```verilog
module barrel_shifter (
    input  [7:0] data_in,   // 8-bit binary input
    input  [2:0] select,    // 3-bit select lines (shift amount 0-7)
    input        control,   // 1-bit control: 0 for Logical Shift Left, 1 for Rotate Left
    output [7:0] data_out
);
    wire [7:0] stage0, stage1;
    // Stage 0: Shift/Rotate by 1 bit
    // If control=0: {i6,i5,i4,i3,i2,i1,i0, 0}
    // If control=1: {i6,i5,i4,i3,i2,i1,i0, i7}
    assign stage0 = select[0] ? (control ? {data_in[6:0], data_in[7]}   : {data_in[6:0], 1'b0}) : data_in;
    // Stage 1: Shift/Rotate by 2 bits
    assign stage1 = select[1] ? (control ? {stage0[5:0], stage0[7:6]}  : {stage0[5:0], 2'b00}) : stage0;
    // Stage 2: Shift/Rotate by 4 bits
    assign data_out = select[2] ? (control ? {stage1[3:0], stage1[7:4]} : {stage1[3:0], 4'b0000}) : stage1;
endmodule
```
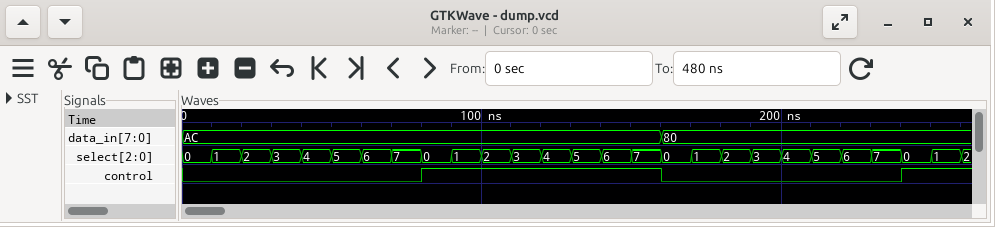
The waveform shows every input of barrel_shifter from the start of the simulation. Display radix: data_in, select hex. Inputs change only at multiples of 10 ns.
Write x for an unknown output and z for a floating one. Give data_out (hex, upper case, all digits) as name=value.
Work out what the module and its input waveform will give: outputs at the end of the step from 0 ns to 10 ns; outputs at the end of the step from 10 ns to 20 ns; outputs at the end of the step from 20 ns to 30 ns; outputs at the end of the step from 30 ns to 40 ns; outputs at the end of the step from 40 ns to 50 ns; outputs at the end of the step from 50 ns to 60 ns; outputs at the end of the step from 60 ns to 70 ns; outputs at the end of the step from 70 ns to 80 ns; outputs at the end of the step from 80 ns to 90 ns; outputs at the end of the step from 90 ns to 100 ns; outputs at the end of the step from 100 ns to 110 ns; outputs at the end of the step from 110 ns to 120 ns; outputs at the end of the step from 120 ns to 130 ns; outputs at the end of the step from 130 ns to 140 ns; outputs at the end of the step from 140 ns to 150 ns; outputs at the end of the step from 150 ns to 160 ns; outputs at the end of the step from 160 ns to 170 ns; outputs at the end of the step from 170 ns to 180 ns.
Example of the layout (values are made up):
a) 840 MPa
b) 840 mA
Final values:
a) data_out=AC
b) data_out=58
c) data_out=B0
d) data_out=60
e) data_out=C0
f) data_out=80
g) data_out=00
h) data_out=00
i) data_out=AC
j) data_out=59
k) data_out=B2
l) data_out=65
m) data_out=CA
n) data_out=95
o) data_out=2B
p) data_out=56
q) data_out=80
r) data_out=00
